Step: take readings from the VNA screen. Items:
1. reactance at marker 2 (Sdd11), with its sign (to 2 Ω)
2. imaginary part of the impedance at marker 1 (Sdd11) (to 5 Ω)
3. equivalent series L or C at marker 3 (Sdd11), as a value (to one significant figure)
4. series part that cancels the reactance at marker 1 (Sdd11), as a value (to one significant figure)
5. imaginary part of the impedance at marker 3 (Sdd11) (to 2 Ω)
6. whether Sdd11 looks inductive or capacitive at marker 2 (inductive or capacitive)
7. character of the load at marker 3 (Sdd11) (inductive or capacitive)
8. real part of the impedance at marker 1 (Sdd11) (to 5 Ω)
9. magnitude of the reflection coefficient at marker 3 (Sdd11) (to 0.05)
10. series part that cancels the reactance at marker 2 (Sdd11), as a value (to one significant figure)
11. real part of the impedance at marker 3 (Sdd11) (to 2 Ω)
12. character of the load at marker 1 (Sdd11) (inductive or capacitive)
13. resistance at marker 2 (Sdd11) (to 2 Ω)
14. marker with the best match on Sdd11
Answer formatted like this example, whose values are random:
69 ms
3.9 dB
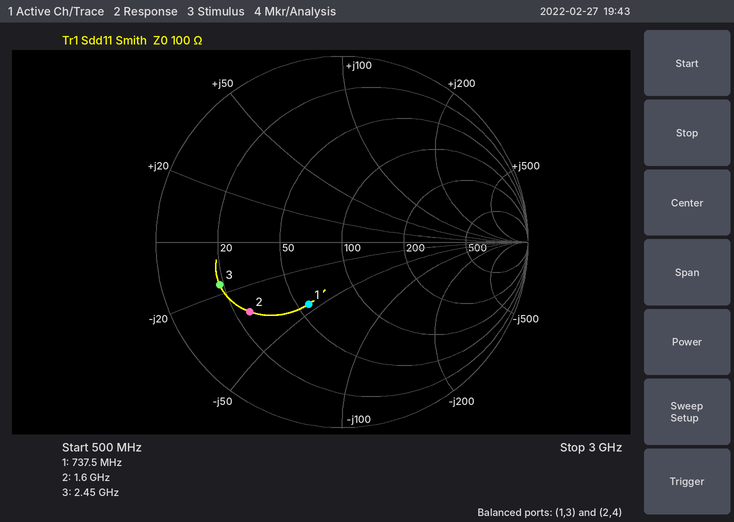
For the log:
-32 Ω
-45 Ω
4 pF
10 nH
-16 Ω
capacitive
capacitive
55 Ω
0.70
3 nH
18 Ω
capacitive
26 Ω
marker 1
